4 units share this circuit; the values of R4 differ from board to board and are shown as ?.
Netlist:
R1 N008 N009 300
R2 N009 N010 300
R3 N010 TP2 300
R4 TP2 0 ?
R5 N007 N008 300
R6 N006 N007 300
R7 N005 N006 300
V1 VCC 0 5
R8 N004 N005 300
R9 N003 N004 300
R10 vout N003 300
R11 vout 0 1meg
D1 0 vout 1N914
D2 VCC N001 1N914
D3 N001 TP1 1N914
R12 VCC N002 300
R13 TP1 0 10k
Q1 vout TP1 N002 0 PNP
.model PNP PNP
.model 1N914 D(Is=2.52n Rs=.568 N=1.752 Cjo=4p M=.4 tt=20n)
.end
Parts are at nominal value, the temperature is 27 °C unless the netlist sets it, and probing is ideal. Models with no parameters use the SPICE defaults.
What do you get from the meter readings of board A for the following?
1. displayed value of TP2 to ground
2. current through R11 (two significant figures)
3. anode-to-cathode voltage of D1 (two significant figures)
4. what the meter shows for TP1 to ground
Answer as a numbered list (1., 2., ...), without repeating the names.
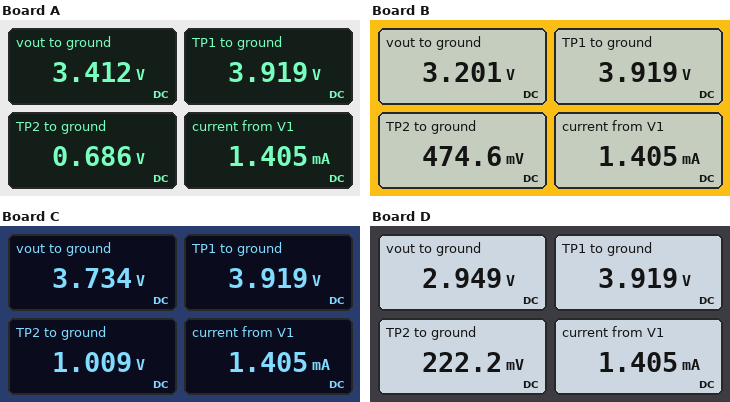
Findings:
1. 0.686 V
2. 3.4 µA
3. -3.4 V
4. 3.919 V
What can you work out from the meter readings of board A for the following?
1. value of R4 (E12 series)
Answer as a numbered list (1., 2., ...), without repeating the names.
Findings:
1. 680 Ω
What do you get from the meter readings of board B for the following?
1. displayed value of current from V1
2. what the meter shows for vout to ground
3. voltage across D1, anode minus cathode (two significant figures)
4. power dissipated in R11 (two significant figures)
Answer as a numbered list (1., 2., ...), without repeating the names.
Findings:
1. 1.405 mA
2. 3.201 V
3. -3.2 V
4. 10 µW
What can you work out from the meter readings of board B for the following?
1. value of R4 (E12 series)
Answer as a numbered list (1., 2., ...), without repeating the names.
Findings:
1. 470 Ω
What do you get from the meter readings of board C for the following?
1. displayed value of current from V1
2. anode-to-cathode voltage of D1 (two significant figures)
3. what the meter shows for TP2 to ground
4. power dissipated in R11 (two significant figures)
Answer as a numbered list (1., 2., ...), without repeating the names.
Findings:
1. 1.405 mA
2. -3.7 V
3. 1.009 V
4. 14 µW
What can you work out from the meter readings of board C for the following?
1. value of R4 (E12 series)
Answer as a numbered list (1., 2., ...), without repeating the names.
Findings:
1. 1 kΩ
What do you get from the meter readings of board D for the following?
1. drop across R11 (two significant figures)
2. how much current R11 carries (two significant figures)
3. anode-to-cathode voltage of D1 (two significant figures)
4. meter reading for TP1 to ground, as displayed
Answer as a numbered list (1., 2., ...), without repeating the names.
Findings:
1. 2.9 V
2. 2.9 µA
3. -2.9 V
4. 3.919 V
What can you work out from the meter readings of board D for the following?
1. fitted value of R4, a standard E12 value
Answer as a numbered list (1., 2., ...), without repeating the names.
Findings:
1. 220 Ω
